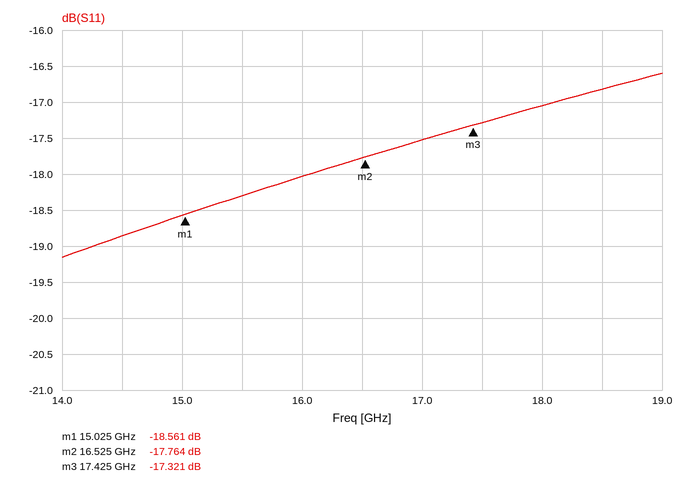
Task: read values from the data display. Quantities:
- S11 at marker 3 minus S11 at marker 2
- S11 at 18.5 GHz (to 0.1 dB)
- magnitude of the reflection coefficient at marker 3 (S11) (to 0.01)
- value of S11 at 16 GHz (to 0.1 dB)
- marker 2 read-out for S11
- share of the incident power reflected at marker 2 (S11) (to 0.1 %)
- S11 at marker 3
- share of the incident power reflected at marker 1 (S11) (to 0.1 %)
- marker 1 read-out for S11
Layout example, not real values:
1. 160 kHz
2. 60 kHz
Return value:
1. 0.443 dB
2. -16.8 dB
3. 0.14
4. -18.0 dB
5. -17.764 dB
6. 1.7 %
7. -17.321 dB
8. 1.4 %
9. -18.561 dB
